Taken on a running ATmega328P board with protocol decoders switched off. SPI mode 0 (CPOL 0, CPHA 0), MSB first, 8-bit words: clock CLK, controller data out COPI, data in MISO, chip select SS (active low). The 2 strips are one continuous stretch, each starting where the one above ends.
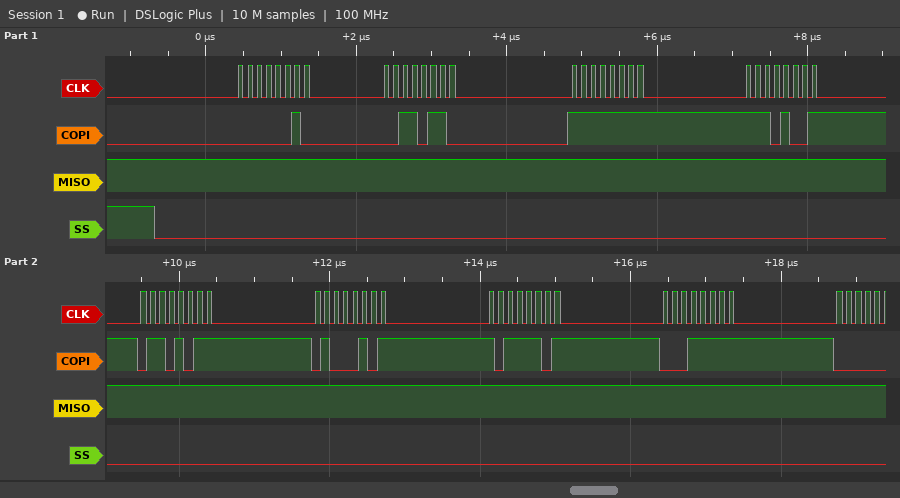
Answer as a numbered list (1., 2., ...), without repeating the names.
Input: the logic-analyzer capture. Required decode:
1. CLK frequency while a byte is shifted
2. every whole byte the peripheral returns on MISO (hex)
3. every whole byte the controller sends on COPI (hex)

1. 8 MHz
2. FF FF FF FF FF FF FF FF
3. 02 36 FF E9 6B 45 BD 1F
